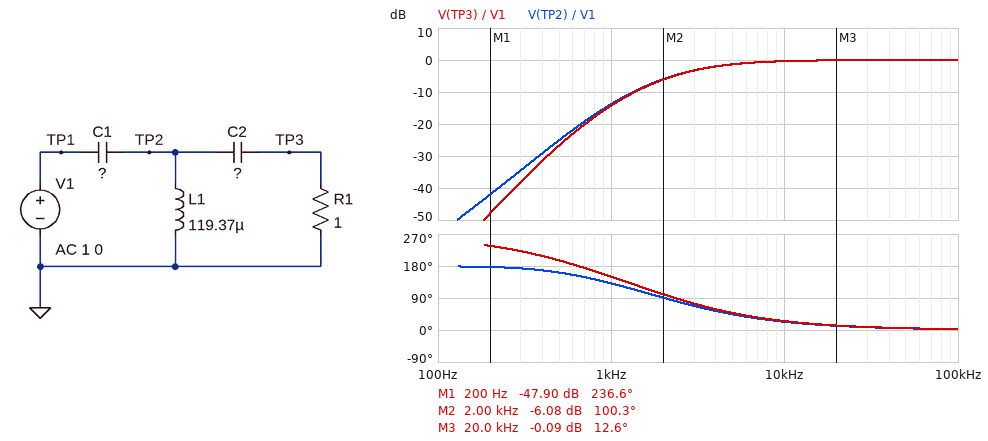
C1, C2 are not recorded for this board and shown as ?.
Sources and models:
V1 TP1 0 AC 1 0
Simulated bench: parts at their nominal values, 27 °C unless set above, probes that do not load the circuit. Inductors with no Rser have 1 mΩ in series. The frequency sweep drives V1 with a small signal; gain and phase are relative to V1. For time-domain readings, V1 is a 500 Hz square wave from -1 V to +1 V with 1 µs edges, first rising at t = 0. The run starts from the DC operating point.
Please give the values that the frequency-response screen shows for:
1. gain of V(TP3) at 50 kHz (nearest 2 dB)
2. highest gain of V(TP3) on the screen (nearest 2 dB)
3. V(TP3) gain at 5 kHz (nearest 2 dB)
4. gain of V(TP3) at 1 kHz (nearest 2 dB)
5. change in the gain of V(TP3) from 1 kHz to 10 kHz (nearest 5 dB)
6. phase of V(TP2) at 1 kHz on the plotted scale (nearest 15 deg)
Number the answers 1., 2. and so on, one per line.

1. 0 dB
2. 0 dB
3. -2 dB
4. -14 dB
5. 15 dB
6. 135 deg
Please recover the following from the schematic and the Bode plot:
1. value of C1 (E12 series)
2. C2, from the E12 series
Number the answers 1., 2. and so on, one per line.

1. 39 µF
2. 470 µF
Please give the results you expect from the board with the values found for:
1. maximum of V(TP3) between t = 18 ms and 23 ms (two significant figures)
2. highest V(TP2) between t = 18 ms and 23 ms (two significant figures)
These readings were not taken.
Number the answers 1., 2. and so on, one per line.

1. 2.0 V
2. 2.0 V
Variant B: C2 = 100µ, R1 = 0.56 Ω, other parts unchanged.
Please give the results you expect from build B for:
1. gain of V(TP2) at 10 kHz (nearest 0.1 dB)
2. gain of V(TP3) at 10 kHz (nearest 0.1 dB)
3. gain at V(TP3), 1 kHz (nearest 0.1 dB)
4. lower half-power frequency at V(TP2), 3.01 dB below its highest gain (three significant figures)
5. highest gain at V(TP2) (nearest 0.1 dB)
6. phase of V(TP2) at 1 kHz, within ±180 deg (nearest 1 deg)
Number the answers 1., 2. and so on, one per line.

1. -2.4 dB
2. -2.8 dB
3. -16.8 dB
4. 1.13 kHz
5. 0.2 dB
6. 159 deg
